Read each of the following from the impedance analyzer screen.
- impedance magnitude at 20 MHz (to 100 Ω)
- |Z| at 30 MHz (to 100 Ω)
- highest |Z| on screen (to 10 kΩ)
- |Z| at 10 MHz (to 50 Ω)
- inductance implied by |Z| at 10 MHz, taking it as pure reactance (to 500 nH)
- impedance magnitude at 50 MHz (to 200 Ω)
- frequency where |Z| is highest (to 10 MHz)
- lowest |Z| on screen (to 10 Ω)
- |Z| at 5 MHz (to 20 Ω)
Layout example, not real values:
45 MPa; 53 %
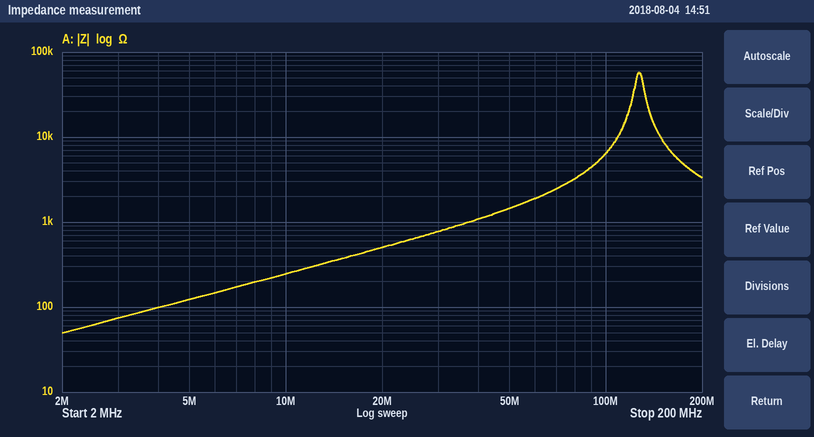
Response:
500 Ω; 800 Ω; 60 kΩ; 250 Ω; 4.0 µH; 1.4 kΩ; 130 MHz; 50 Ω; 120 Ω
